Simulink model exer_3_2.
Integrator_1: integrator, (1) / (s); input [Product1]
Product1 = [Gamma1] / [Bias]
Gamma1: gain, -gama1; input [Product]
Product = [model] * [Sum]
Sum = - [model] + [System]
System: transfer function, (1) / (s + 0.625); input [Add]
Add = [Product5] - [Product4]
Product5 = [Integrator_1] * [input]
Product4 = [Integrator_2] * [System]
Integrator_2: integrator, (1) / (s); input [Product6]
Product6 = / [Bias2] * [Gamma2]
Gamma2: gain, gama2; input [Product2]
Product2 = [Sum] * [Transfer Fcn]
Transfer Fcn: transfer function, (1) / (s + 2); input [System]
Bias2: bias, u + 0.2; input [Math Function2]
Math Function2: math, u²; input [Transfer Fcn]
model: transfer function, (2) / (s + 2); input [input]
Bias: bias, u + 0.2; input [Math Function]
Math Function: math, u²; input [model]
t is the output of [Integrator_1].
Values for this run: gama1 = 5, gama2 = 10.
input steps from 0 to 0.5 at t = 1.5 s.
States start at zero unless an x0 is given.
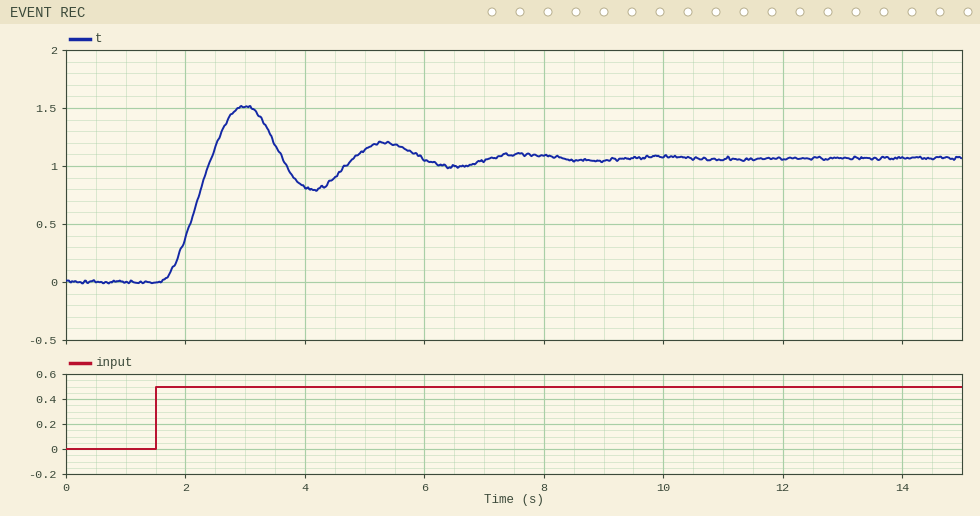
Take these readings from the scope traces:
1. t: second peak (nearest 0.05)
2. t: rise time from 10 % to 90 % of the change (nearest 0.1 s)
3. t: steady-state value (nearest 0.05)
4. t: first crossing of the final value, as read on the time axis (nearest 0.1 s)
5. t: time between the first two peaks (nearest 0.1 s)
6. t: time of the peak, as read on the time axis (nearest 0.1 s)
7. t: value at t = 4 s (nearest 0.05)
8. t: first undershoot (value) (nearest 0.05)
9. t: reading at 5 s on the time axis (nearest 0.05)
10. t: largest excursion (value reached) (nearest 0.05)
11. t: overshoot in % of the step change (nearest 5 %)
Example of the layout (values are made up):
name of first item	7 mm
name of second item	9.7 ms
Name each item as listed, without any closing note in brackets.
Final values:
t: second peak	1.20
t: rise time from 10 % to 90 % of the change	0.6 s
t: steady-state value	1.05
t: first crossing of the final value, as read on the time axis	2.4 s
t: time between the first two peaks	2.3 s
t: time of the peak, as read on the time axis	3.0 s
t: value at t = 4 s	0.80
t: first undershoot (value)	0.80
t: reading at 5 s on the time axis	1.15
t: largest excursion (value reached)	1.50
t: overshoot in % of the step change	40 %
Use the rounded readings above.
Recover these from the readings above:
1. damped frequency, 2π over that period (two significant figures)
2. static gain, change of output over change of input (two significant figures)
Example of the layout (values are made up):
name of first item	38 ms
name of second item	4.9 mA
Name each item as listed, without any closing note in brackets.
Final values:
damped frequency, 2π over that period	2.7 rad/s
static gain, change of output over change of input	2.1
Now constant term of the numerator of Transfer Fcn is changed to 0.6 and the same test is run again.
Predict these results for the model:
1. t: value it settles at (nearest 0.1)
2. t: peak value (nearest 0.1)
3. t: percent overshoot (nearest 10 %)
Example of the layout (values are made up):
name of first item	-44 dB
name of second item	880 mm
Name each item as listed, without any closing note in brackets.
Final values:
t: value it settles at	1.0
t: peak value	1.5
t: percent overshoot	50 %
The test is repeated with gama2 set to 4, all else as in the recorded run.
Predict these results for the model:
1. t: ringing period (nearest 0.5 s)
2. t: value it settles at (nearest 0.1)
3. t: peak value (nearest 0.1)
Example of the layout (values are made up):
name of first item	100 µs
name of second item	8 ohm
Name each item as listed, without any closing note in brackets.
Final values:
t: ringing period	3.0 s
t: value it settles at	0.9
t: peak value	1.5
